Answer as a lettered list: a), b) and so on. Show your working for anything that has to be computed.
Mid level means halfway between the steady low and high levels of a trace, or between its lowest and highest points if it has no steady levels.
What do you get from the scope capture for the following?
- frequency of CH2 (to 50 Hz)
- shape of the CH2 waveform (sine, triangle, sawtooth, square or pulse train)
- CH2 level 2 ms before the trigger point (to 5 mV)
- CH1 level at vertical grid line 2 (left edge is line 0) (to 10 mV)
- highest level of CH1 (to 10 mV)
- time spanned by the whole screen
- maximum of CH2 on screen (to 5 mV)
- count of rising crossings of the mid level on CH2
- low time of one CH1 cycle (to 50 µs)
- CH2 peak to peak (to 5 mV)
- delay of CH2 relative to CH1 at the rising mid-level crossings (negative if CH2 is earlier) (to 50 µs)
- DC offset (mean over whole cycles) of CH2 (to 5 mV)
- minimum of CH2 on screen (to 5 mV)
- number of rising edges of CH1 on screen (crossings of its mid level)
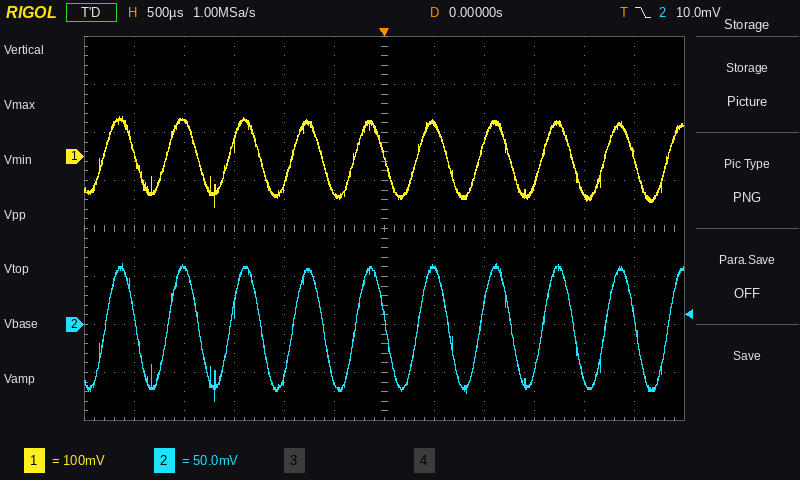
a) 1.60 kHz
b) sine
c) 60 mV
d) 70 mV
e) 80 mV
f) 6 ms
g) 65 mV
h) 10
i) 300 µs
j) 65 mV − (-80 mV) = 145 mV
k) 0 µs
l) (65 mV + (-80 mV)) / 2 ≈ -7.50 mV, so -5 mV to the nearest 5 mV
m) -80 mV
n) 10
